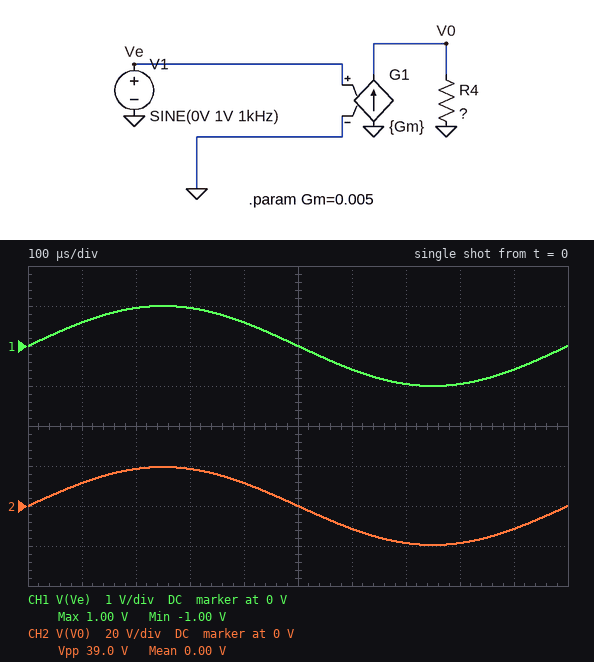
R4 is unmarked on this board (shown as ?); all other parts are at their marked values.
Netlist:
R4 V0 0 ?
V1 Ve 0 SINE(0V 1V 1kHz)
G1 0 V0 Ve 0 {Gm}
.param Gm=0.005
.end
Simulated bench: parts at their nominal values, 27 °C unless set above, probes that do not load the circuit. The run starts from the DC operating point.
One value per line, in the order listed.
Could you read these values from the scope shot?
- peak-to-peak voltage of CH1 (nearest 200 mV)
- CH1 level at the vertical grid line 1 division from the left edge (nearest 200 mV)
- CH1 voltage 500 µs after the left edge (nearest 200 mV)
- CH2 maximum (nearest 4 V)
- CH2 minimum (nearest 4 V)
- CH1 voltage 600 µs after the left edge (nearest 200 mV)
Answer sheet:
2.0 V
600 mV
0 V
20 V
-20 V
-600 mV
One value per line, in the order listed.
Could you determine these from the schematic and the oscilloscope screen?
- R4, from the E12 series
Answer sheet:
3.9 kΩ
